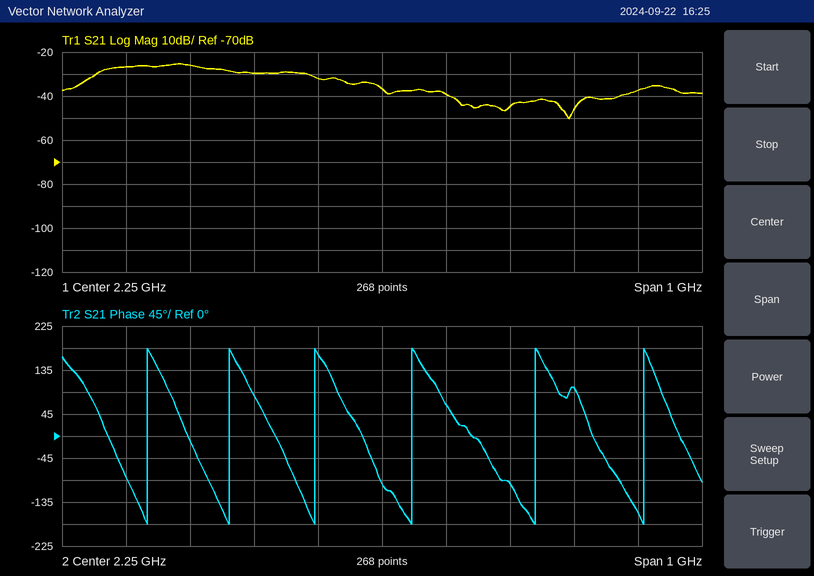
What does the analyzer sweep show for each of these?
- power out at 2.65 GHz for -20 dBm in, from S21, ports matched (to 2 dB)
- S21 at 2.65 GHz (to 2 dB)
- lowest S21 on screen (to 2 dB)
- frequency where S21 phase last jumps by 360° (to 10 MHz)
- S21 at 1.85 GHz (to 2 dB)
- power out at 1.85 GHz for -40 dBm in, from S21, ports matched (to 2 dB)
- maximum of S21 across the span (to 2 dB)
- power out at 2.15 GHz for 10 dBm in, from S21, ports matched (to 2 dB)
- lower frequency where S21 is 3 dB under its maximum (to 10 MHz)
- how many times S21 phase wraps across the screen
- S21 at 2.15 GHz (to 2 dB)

-58 dBm
-38 dB
-50 dB
2.66 GHz
-26 dB
-66 dBm
-26 dB
-22 dBm
1.81 GHz
6
-32 dB
